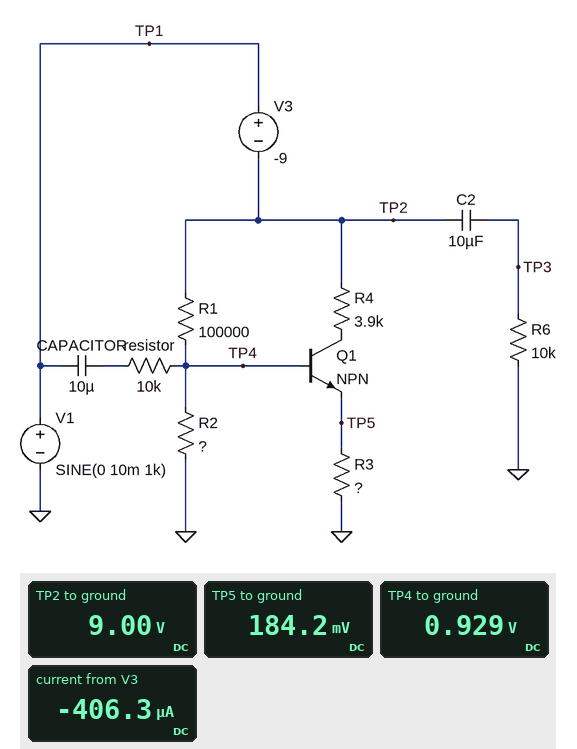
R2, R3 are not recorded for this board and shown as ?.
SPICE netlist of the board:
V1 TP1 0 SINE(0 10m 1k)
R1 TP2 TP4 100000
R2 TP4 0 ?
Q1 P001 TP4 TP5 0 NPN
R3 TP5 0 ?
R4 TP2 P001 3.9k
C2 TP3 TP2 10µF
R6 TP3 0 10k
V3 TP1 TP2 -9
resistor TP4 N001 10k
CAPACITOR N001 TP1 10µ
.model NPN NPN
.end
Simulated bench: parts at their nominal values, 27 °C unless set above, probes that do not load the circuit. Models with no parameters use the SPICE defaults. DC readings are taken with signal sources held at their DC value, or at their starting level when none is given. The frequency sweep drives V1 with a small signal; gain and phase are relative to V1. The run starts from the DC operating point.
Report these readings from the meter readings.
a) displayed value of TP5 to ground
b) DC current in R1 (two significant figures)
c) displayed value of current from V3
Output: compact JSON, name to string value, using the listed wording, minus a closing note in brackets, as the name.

{"displayed value of TP5 to ground": "184.2 mV", "DC current in R1": "81 µA", "displayed value of current from V3": "-406.3 µA"}
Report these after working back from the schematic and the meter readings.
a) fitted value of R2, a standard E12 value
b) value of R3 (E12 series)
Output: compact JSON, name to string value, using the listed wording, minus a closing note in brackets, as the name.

{"fitted value of R2, a standard E12 value": "12 kΩ", "value of R3": "560 Ω"}
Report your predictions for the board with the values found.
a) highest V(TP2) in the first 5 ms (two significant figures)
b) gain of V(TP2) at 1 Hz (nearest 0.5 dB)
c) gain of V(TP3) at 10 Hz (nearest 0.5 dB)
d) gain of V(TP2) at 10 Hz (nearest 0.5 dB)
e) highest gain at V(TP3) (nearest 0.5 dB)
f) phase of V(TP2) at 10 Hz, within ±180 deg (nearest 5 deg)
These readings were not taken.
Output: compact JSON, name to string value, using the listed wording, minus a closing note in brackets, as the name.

{"highest V(TP2) in the first 5 ms": "9.0 V", "gain of V(TP2) at 1 Hz": "0 dB", "gain of V(TP3) at 10 Hz": "0 dB", "gain of V(TP2) at 10 Hz": "0 dB", "highest gain at V(TP3)": "0 dB", "phase of V(TP2) at 10 Hz, within ±180 deg": "0 deg"}
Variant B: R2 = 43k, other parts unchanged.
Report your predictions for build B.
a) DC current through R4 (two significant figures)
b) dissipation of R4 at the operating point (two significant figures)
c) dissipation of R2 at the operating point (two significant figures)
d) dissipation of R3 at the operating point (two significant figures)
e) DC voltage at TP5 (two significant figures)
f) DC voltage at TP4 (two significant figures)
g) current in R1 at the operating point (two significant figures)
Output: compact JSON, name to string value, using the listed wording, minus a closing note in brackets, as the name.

{"DC current through R4": "2.0 mA", "dissipation of R4 at the operating point": "15 mW", "dissipation of R2 at the operating point": "85 µW", "dissipation of R3 at the operating point": "2.3 mW", "DC voltage at TP5": "1.1 V", "DC voltage at TP4": "1.9 V", "current in R1 at the operating point": "71 µA"}
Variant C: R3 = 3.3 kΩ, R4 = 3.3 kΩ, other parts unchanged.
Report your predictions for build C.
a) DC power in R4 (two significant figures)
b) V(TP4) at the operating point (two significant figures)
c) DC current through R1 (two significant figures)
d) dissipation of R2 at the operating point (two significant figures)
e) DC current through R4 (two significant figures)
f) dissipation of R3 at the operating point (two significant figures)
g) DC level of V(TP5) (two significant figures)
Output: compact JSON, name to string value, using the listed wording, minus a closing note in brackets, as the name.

{"DC power in R4": "18 µW", "V(TP4) at the operating point": "960 mV", "DC current through R1": "80 µA", "dissipation of R2 at the operating point": "76 µW", "DC current through R4": "75 µA", "dissipation of R3 at the operating point": "19 µW", "DC level of V(TP5)": "250 mV"}
